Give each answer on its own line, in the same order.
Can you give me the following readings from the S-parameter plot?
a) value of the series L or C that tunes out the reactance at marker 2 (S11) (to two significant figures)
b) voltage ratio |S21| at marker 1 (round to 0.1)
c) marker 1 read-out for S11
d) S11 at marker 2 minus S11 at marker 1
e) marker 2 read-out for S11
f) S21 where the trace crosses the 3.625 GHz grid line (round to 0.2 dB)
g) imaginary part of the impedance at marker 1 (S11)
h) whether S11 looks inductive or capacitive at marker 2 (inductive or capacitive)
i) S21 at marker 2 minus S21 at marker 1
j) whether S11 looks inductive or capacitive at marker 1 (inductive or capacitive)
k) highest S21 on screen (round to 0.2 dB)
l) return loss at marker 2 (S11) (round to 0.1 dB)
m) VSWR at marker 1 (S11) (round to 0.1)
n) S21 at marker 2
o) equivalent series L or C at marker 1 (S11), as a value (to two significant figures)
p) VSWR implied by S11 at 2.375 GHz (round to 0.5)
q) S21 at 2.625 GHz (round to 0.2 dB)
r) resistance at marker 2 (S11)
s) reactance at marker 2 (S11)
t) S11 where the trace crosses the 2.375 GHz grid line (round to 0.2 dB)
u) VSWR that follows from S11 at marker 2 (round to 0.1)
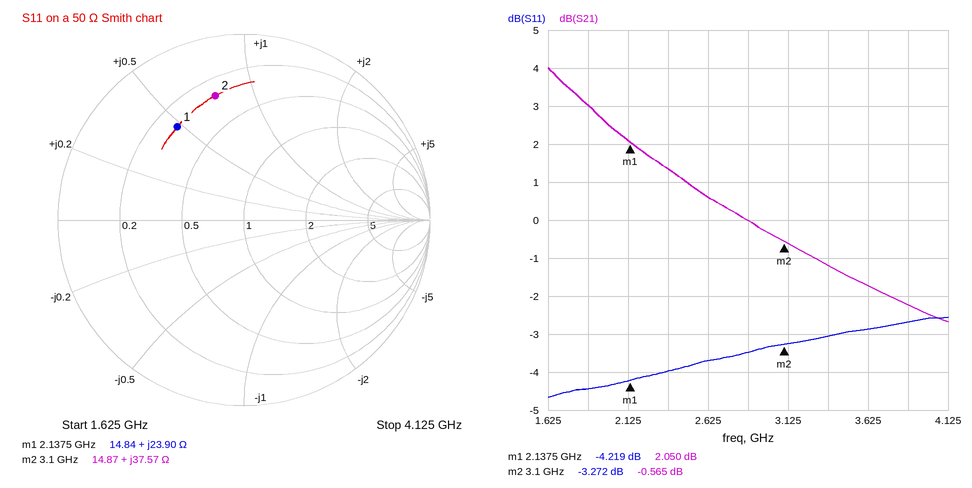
1.4 pF
1.3
-4.219 dB
0.947 dB
-3.272 dB
-1.8 dB
+23.90 Ω
inductive
-2.615 dB
inductive
4.0 dB
3.3 dB
4.2
-0.565 dB
1.8 nH
4.5
0.6 dB
14.87 Ω
+37.57 Ω
-4.0 dB
5.4
